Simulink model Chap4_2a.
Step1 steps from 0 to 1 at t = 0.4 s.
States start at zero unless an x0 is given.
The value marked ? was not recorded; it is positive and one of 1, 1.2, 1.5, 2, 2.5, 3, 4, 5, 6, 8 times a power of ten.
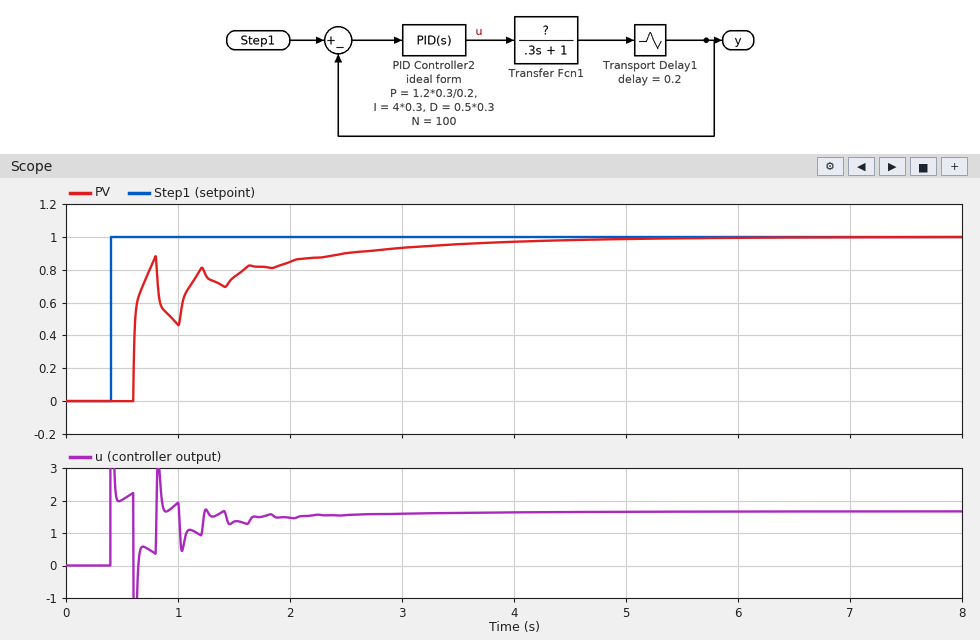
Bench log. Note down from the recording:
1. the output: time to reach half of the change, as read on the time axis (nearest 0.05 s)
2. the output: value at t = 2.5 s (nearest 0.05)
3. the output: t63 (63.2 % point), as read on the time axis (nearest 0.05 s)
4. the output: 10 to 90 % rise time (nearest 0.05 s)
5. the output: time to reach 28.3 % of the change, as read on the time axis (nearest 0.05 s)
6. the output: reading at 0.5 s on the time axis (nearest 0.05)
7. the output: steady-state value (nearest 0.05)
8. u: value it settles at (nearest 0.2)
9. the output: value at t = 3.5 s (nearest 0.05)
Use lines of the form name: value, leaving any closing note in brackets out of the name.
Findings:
the output: time to reach half of the change, as read on the time axis: 0.60 s
the output: value at t = 2.5 s: 0.90
the output: t63 (63.2 % point), as read on the time axis: 0.65 s
the output: 10 to 90 % rise time: 1.90 s
the output: time to reach 28.3 % of the change, as read on the time axis: 0.60 s
the output: reading at 0.5 s on the time axis: 0.00
the output: steady-state value: 1.00
u: value it settles at: 1.6
the output: value at t = 3.5 s: 0.95
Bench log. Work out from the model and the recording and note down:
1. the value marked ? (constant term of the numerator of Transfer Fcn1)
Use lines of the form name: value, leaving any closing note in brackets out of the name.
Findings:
the value marked ?: 0.6
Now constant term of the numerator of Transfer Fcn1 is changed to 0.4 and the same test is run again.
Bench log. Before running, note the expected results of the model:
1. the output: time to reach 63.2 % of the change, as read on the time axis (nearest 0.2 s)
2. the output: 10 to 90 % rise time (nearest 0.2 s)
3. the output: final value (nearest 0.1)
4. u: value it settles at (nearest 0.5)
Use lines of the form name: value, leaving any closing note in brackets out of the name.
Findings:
the output: time to reach 63.2 % of the change, as read on the time axis: 1.4 s
the output: 10 to 90 % rise time: 2.8 s
the output: final value: 1.0
u: value it settles at: 2.5
